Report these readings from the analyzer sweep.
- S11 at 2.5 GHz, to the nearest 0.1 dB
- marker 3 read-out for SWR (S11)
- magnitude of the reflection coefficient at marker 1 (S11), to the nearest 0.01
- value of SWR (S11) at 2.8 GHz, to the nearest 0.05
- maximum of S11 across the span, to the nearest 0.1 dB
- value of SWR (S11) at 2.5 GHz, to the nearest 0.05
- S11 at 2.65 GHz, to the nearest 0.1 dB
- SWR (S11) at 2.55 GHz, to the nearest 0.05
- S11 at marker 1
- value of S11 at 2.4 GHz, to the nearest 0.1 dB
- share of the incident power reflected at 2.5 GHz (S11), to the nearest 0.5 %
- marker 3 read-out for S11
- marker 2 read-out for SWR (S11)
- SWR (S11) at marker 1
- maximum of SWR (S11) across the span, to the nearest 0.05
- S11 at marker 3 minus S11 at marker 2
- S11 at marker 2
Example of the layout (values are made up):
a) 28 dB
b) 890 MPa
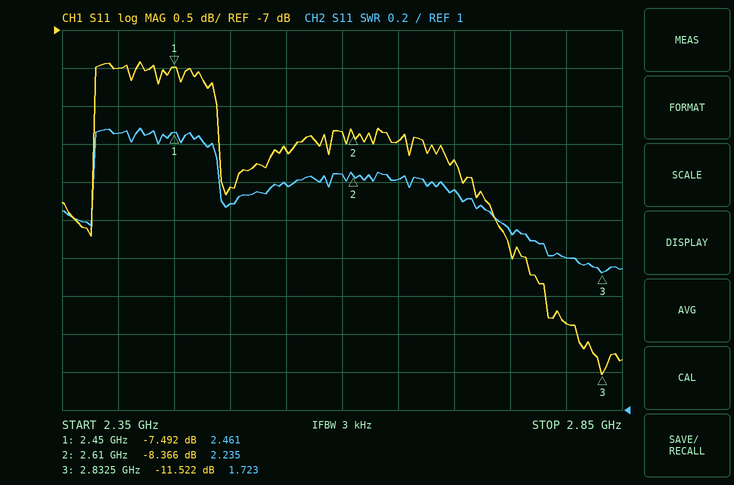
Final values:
a) -9.1 dB
b) 1.723
c) 0.42
d) 1.80
e) -7.4 dB
f) 2.10
g) -8.5 dB
h) 2.20
i) -7.492 dB
j) -7.5 dB
k) 12.5 %
l) -11.522 dB
m) 2.235
n) 2.461
o) 2.50
p) -3.156 dB
q) -8.366 dB
